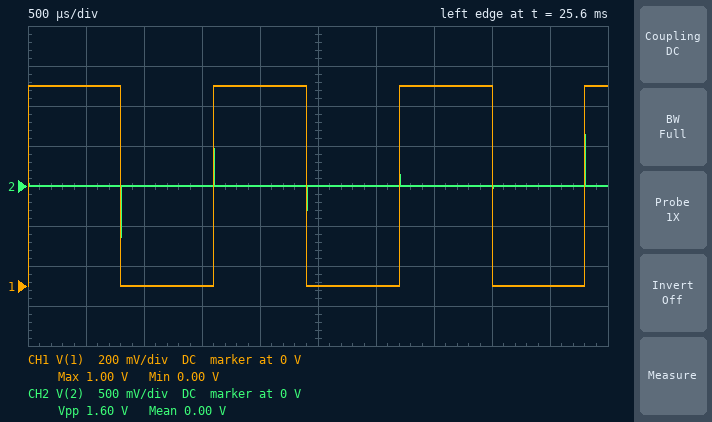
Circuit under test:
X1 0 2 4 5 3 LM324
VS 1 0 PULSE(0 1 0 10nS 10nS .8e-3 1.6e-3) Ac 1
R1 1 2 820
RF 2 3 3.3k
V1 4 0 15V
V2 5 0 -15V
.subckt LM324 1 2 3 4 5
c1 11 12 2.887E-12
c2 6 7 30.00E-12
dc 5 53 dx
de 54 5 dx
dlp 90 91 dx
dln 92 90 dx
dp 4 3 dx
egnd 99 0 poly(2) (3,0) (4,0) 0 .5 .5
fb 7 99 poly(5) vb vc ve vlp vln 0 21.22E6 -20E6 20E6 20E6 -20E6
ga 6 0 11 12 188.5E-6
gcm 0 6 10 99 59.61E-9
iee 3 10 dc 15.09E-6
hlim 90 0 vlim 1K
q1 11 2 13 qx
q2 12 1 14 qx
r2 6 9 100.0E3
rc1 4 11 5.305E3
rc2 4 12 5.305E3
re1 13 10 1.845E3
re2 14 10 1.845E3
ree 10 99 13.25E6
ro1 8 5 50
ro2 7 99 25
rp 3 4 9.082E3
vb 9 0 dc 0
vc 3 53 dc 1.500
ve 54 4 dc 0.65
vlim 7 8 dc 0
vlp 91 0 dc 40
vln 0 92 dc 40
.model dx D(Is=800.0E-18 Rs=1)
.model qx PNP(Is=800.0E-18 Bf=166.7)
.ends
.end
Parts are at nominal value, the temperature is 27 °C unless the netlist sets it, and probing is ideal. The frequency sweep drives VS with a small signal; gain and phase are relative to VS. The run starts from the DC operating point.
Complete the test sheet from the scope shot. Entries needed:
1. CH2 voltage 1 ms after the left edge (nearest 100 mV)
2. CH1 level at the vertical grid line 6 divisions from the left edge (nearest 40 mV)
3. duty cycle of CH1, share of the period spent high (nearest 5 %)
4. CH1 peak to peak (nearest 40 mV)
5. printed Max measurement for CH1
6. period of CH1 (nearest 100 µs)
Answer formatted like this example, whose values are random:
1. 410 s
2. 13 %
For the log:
1. 0 V
2. 0 V
3. 50 %
4. 1.00 V
5. 1.00 V
6. 1.6 ms
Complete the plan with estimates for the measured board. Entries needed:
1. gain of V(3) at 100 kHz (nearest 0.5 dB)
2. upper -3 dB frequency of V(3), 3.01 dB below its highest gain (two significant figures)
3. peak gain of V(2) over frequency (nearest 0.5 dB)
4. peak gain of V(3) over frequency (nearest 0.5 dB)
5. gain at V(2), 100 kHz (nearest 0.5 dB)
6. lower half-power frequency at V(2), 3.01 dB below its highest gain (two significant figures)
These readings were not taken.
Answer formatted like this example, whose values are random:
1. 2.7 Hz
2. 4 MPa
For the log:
1. 11.0 dB
2. 200 kHz
3. -1.5 dB
4. 12.0 dB
5. -8.5 dB
6. 200 kHz
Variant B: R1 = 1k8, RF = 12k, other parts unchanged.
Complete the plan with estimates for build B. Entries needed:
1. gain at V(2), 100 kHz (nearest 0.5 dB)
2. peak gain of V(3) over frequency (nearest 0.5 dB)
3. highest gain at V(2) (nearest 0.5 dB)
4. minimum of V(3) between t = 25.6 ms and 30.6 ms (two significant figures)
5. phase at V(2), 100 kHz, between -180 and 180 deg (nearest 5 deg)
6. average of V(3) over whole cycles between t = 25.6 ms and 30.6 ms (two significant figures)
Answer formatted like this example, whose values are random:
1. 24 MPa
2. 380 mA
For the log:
1. -5.5 dB
2. 16.5 dB
3. -1.0 dB
4. -6.7 V
5. 55 deg
6. -3.3 V
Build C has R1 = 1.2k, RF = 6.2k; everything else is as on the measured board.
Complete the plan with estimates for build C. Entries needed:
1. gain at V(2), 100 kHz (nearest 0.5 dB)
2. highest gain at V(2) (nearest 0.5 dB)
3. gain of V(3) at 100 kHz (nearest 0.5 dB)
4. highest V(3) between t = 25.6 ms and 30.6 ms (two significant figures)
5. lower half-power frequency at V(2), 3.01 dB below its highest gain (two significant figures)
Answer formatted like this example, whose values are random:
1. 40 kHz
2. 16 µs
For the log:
1. -7.0 dB
2. -1.5 dB
3. 13.0 dB
4. 4.6 mV
5. 160 kHz
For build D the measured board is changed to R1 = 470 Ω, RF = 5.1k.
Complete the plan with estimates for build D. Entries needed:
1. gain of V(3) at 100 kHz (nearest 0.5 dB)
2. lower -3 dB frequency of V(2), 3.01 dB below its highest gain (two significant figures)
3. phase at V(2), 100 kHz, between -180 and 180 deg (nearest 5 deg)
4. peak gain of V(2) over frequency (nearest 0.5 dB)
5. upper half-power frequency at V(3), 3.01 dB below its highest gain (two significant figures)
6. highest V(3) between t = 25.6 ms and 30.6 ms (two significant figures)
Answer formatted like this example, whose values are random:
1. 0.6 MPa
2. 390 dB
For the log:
1. 17.0 dB
2. 84 kHz
3. 40 deg
4. -0.5 dB
5. 85 kHz
6. 5.7 mV
